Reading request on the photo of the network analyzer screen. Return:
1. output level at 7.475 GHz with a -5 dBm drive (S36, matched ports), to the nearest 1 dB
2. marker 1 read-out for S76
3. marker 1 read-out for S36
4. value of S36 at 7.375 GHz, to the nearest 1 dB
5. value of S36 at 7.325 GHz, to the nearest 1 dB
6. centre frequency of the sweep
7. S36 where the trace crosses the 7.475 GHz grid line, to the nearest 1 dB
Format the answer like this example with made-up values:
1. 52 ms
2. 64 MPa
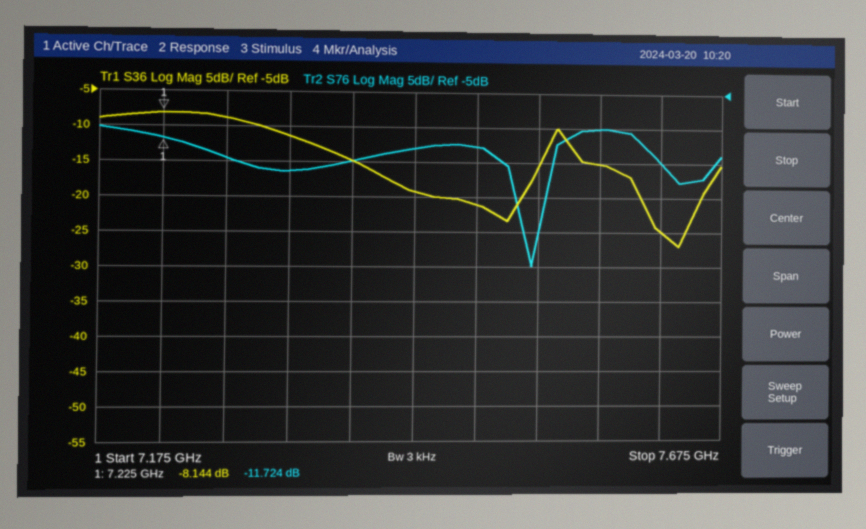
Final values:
1. -26 dBm
2. -11.724 dB
3. -8.144 dB
4. -15 dB
5. -11 dB
6. 7.425 GHz
7. -21 dB
